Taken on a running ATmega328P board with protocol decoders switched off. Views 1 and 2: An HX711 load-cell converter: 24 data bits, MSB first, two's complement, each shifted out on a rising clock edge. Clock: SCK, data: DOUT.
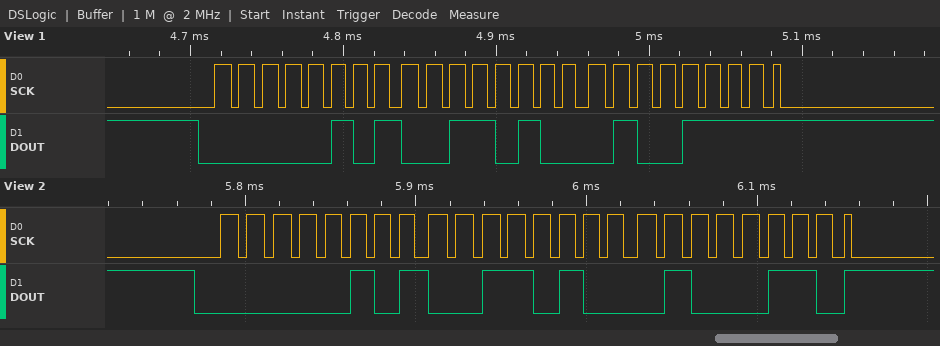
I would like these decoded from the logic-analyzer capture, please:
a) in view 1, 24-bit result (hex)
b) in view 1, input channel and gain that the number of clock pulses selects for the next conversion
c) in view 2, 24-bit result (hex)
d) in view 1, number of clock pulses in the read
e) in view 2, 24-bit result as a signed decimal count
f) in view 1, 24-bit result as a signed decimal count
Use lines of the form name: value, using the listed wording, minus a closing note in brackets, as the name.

in view 1, 24-bit result: 0x05344F
in view 1, input channel and gain that the number of clock pulses selects for the next conversion: channel A, gain 128
in view 2, 24-bit result: 0x053446
in view 1, number of clock pulses in the read: 25
in view 2, 24-bit result as a signed decimal count: 341062
in view 1, 24-bit result as a signed decimal count: 341071
